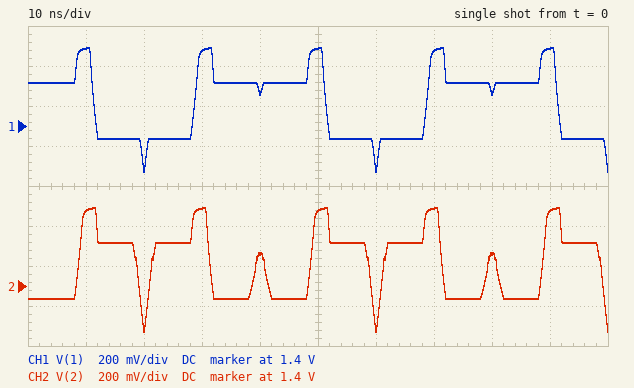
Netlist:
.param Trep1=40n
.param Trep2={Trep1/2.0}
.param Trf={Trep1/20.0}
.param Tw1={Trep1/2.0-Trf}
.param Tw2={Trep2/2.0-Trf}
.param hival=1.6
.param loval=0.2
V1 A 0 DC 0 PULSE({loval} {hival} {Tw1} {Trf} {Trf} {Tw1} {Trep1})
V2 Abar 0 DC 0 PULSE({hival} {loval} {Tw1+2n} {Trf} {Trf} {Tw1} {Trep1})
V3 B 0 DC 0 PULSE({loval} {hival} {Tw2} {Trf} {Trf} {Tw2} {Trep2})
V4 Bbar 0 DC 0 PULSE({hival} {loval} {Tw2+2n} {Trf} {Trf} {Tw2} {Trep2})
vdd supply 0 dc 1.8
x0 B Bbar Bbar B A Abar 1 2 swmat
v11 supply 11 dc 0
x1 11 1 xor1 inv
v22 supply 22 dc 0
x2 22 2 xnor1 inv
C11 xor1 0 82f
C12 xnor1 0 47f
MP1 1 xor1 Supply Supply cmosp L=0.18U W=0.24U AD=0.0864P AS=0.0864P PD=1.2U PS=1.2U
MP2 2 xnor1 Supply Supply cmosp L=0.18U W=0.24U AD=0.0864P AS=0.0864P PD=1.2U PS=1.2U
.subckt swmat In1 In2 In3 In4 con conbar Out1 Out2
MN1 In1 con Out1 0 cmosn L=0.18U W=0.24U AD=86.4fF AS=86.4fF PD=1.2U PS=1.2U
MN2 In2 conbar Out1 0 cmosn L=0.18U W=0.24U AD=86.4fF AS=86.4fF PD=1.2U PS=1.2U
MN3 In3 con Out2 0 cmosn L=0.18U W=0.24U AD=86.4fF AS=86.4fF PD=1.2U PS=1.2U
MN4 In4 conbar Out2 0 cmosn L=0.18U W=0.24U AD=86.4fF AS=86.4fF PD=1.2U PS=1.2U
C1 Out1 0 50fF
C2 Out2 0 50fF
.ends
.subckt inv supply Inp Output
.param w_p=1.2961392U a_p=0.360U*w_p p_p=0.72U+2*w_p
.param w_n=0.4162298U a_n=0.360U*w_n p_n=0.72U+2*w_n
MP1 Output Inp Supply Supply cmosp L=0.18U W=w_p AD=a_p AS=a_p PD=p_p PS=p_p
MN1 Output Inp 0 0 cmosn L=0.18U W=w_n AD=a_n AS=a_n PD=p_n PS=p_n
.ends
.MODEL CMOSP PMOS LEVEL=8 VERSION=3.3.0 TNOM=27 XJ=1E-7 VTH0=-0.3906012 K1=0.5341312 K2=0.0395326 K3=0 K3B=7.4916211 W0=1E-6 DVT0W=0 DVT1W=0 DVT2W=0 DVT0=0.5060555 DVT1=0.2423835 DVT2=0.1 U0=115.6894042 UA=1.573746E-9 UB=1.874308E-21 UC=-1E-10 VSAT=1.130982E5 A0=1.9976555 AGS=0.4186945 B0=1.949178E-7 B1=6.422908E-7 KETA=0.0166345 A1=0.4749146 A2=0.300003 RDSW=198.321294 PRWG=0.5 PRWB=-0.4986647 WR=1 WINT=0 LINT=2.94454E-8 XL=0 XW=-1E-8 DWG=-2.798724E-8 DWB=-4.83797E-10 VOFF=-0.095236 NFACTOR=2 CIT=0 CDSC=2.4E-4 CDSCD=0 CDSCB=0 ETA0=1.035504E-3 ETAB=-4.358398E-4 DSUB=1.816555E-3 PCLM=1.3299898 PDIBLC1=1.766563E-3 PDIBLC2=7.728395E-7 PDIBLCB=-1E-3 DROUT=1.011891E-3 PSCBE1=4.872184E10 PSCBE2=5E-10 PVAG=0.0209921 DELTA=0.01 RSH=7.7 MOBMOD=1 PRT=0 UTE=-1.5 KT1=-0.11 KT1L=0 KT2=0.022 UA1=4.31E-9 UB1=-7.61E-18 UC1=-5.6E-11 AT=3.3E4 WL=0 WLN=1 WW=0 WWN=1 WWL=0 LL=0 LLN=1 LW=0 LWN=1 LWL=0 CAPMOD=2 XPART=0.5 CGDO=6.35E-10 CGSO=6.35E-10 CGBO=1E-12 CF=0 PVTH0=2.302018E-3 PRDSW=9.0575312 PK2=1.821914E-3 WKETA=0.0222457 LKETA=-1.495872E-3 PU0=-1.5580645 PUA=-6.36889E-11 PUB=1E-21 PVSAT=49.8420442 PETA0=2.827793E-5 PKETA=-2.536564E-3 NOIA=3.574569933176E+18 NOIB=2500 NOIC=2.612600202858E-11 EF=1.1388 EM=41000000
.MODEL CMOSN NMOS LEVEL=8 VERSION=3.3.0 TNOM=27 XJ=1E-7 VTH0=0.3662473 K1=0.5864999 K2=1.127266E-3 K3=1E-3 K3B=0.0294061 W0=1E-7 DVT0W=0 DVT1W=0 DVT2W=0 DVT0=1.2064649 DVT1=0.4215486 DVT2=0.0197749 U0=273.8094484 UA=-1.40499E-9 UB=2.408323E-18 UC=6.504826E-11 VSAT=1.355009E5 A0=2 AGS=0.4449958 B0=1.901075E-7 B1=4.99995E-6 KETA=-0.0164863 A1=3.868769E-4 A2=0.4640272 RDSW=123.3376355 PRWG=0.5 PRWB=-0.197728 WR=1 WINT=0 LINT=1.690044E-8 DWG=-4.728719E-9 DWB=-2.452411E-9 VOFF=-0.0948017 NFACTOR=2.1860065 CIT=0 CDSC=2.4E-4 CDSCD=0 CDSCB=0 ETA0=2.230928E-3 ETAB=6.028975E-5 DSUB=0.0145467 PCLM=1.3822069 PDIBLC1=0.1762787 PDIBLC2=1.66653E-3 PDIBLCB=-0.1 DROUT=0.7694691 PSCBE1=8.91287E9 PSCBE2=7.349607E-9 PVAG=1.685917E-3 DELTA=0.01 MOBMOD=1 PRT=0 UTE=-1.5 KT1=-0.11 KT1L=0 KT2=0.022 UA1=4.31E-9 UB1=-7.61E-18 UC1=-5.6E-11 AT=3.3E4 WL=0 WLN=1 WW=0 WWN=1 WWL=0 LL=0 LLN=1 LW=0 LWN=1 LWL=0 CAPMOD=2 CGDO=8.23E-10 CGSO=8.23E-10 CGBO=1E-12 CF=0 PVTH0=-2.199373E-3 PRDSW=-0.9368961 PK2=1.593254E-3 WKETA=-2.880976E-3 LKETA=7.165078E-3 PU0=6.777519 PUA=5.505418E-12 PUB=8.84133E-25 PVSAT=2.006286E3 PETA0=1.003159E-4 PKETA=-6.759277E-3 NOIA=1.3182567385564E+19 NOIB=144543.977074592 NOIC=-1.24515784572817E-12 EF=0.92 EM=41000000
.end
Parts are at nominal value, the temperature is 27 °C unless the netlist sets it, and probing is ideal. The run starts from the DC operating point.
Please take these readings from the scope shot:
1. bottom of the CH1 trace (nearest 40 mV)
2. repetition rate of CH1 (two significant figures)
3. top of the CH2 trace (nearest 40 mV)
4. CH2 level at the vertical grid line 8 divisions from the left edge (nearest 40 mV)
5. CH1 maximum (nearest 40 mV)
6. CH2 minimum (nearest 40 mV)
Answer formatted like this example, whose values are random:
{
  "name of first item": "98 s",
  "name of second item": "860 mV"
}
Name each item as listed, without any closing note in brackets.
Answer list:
{
  "bottom of the CH1 trace": "1.16 V",
  "repetition rate of CH1": "25 MHz",
  "top of the CH2 trace": "1.80 V",
  "CH2 level at the vertical grid line 8 divisions from the left edge": "1.56 V",
  "CH1 maximum": "1.80 V",
  "CH2 minimum": "1.16 V"
}
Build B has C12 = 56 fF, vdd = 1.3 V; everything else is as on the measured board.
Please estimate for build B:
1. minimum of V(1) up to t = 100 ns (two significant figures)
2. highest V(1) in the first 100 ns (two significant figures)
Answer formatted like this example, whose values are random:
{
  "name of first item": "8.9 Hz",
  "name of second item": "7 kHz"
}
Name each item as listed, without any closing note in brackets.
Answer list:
{
  "minimum of V(1) up to t = 100 ns": "800 mV",
  "highest V(1) in the first 100 ns": "1.3 V"
}
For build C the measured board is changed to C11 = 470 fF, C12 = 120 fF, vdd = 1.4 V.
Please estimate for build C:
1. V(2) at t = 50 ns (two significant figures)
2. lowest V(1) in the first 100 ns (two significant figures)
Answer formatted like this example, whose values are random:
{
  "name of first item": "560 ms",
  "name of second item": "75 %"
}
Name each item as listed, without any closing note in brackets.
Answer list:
{
  "V(2) at t = 50 ns": "1.4 V",
  "lowest V(1) in the first 100 ns": "870 mV"
}
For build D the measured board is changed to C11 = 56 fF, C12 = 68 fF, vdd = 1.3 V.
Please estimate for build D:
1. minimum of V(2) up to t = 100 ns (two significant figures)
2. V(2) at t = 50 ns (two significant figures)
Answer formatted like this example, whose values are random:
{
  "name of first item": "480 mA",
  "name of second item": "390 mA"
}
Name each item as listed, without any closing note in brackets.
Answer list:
{
  "minimum of V(2) up to t = 100 ns": "800 mV",
  "V(2) at t = 50 ns": "1.3 V"
}
